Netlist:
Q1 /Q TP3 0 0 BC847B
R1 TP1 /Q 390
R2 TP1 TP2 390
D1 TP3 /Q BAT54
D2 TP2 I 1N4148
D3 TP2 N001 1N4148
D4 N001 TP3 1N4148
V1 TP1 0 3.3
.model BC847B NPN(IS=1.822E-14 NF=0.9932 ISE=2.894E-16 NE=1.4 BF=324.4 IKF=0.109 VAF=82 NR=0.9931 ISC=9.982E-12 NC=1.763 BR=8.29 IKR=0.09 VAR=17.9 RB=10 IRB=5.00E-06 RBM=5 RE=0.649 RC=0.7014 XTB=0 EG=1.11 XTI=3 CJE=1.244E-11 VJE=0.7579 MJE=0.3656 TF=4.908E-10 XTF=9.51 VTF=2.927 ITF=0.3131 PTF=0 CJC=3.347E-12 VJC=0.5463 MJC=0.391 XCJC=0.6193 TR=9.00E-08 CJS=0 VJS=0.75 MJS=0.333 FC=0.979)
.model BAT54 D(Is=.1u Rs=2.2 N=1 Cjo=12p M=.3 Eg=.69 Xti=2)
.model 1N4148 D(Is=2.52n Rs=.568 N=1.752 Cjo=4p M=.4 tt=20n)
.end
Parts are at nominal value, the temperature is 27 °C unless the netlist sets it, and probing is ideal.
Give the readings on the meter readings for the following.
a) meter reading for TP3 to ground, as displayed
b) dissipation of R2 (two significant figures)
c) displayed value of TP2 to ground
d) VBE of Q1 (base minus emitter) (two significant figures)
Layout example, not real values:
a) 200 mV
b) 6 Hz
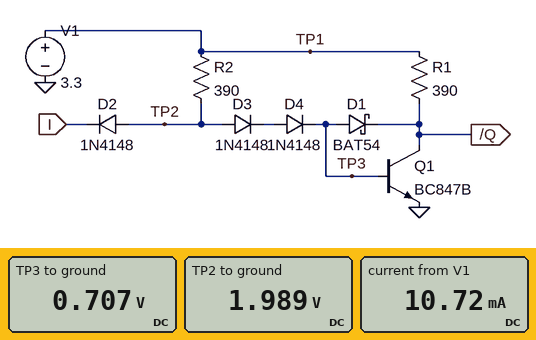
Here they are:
a) 0.707 V
b) 4.4 mW
c) 1.989 V
d) 710 mV
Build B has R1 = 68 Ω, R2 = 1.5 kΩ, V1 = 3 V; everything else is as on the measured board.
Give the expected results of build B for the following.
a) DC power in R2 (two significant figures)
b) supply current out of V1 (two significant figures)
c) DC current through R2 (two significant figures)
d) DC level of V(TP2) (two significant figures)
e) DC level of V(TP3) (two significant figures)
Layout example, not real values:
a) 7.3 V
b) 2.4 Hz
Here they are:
a) 800 µW
b) 37 mA
c) 730 µA
d) 1.9 V
e) 760 mV
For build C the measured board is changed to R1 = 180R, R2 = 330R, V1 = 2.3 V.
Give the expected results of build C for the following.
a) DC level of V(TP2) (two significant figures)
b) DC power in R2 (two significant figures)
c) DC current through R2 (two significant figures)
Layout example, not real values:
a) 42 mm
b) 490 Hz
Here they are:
a) 1.9 V
b) 490 µW
c) 1.2 mA
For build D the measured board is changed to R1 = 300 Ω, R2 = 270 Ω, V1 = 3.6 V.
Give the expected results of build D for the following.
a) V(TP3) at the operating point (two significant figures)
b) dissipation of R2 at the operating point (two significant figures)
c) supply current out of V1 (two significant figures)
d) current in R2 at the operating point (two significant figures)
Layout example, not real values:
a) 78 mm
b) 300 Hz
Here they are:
a) 720 mV
b) 8.8 mW
c) 16 mA
d) 5.7 mA
